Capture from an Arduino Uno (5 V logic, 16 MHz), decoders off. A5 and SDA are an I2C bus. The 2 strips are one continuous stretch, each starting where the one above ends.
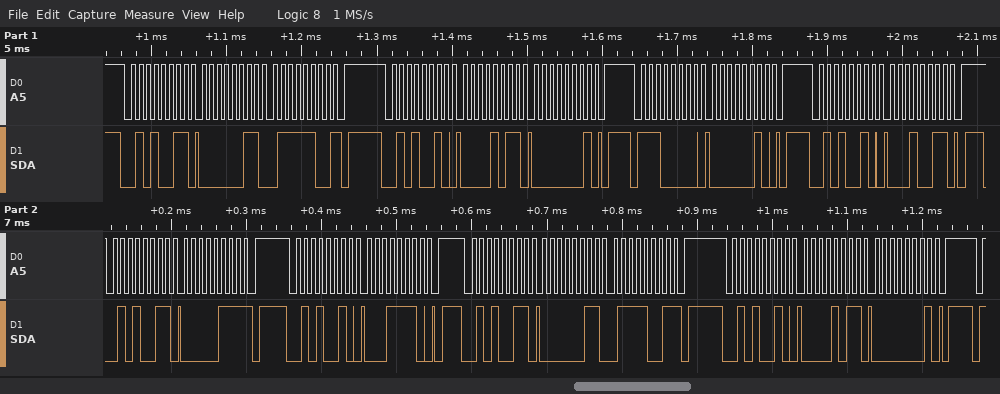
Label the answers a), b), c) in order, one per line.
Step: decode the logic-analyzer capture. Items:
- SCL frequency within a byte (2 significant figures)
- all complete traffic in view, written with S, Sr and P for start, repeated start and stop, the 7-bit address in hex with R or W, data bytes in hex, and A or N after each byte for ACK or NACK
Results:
a) 100 kHz
b) S 29R A 03 A 7C N P S 29W A 0B A 01 A P S 70W A 02 A P S 29W A 13 A P S 29R A 07 N P S 29W A 1E A P S 29R A 03 A 79 N P S 29W A 0B A 01 A P
